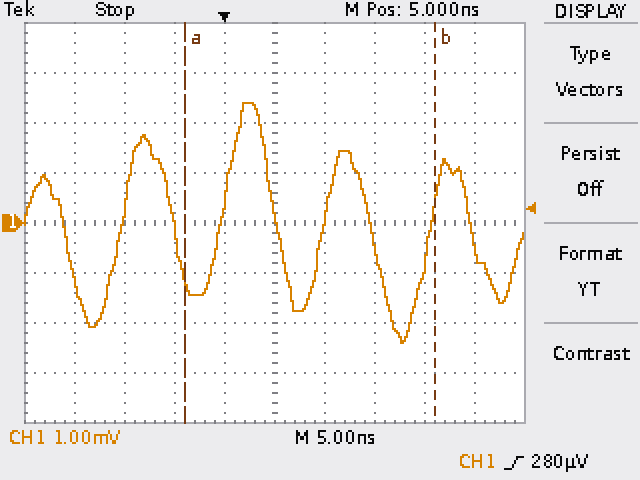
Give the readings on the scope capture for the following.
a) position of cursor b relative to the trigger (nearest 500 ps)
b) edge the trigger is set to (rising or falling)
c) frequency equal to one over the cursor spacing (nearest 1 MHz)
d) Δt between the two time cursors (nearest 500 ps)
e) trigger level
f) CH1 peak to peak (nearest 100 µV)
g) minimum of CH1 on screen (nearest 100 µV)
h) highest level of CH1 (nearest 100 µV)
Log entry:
+21.0 ns
rising
40 MHz
25.0 ns
280 µV
4.8 mV
-2.4 mV
2.4 mV
